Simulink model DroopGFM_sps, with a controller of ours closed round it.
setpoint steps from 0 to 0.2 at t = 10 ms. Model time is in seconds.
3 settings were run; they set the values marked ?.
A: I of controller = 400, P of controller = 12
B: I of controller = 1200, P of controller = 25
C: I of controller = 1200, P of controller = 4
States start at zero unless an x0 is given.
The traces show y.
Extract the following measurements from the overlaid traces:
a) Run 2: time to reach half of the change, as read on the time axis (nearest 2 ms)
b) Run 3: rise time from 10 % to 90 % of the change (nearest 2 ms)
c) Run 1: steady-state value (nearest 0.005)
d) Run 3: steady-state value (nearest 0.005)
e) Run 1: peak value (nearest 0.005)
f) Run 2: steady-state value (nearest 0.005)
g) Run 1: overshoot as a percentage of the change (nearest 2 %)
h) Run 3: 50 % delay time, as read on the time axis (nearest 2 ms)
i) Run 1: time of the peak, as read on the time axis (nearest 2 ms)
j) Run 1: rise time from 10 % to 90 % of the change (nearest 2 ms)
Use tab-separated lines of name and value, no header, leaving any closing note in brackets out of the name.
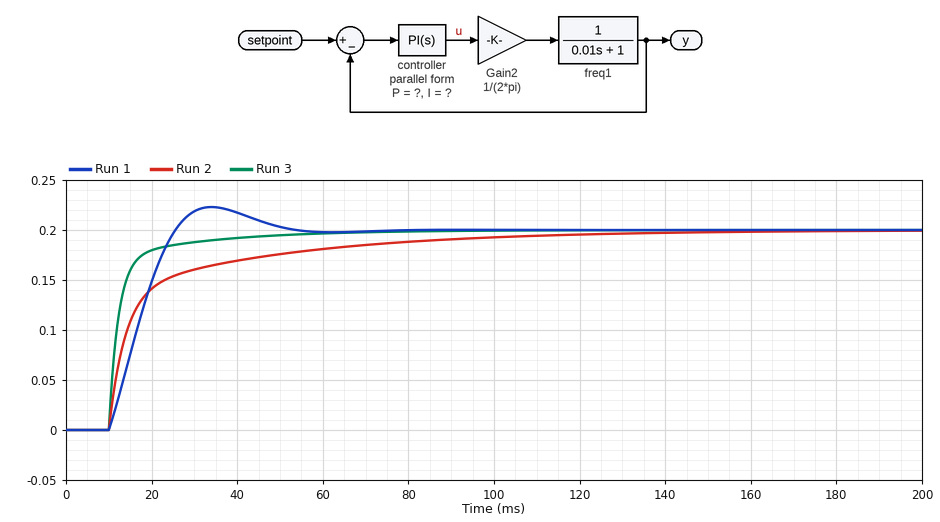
Run 2: time to reach half of the change, as read on the time axis	14 ms
Run 3: rise time from 10 % to 90 % of the change	10 ms
Run 1: steady-state value	0.200
Run 3: steady-state value	0.200
Run 1: peak value	0.225
Run 2: steady-state value	0.200
Run 1: overshoot as a percentage of the change	12 %
Run 3: 50 % delay time, as read on the time axis	12 ms
Run 1: time of the peak, as read on the time axis	34 ms
Run 1: rise time from 10 % to 90 % of the change	12 ms
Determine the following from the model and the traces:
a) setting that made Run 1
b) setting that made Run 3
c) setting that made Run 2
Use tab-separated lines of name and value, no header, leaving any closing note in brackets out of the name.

setting that made Run 1	C
setting that made Run 3	B
setting that made Run 2	A
